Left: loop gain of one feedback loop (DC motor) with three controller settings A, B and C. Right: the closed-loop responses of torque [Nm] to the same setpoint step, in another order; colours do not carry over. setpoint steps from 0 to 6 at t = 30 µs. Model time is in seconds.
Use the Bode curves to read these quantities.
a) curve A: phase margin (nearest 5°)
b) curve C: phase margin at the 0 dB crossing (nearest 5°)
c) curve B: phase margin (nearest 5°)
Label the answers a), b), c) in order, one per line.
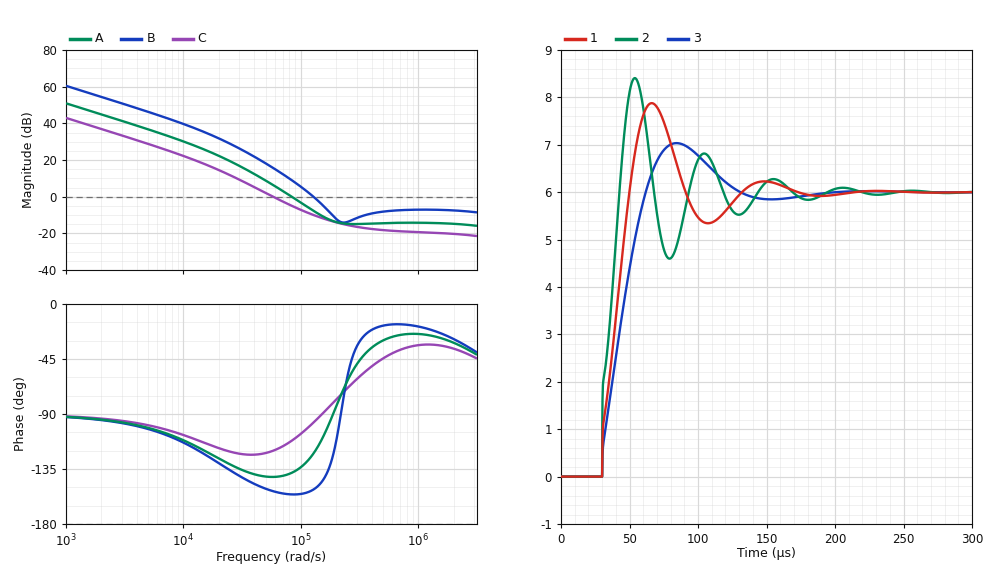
a) 40°
b) 60°
c) 30°
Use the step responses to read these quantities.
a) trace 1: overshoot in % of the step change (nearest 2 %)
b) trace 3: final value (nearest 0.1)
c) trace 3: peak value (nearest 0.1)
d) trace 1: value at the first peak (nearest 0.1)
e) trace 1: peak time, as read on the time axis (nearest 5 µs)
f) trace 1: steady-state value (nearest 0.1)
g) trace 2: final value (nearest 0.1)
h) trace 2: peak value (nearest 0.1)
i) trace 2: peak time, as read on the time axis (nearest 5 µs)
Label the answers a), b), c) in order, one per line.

a) 32 %
b) 6.0
c) 7.0
d) 7.9
e) 65 µs
f) 6.0
g) 6.0
h) 8.4
i) 55 µs
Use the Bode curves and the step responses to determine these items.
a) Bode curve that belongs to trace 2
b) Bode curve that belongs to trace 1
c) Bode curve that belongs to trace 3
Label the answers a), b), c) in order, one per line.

a) B
b) A
c) C
